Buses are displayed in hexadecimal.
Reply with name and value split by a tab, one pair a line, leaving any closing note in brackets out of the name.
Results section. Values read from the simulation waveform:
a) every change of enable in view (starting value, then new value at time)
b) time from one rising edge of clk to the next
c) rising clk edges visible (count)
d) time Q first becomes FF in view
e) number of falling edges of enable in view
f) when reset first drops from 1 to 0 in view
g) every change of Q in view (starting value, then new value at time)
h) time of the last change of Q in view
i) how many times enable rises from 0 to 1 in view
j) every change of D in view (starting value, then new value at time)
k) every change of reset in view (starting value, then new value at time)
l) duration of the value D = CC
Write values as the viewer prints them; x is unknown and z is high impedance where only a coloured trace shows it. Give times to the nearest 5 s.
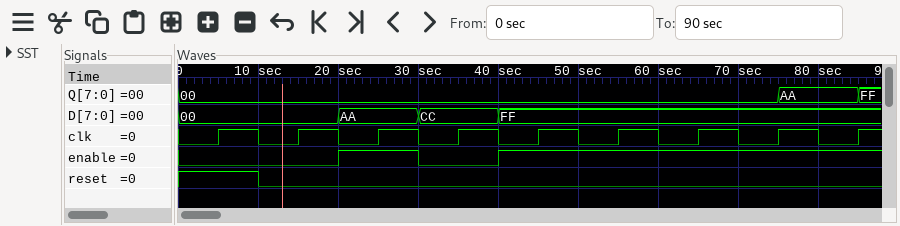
every change of enable in view	0, 1 at 20 s, 0 at 30 s, 1 at 40 s
time from one rising edge of clk to the next	10 s
rising clk edges visible	9
time Q first becomes FF in view	85 s
number of falling edges of enable in view	1
when reset first drops from 1 to 0 in view	10 s
every change of Q in view	00, AA at 75 s, FF at 85 s
time of the last change of Q in view	85 s
how many times enable rises from 0 to 1 in view	2
every change of D in view	00, AA at 20 s, CC at 30 s, FF at 40 s
every change of reset in view	1, 0 at 10 s
duration of the value D = CC	10 s
